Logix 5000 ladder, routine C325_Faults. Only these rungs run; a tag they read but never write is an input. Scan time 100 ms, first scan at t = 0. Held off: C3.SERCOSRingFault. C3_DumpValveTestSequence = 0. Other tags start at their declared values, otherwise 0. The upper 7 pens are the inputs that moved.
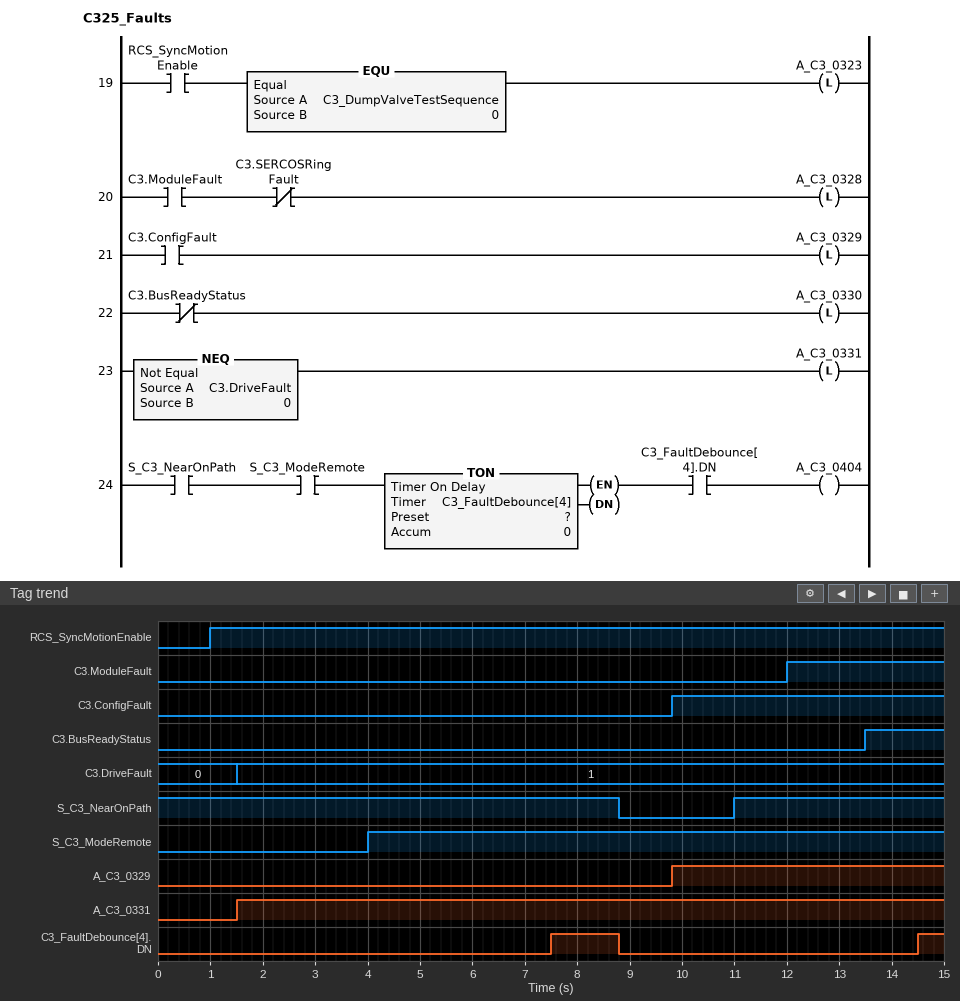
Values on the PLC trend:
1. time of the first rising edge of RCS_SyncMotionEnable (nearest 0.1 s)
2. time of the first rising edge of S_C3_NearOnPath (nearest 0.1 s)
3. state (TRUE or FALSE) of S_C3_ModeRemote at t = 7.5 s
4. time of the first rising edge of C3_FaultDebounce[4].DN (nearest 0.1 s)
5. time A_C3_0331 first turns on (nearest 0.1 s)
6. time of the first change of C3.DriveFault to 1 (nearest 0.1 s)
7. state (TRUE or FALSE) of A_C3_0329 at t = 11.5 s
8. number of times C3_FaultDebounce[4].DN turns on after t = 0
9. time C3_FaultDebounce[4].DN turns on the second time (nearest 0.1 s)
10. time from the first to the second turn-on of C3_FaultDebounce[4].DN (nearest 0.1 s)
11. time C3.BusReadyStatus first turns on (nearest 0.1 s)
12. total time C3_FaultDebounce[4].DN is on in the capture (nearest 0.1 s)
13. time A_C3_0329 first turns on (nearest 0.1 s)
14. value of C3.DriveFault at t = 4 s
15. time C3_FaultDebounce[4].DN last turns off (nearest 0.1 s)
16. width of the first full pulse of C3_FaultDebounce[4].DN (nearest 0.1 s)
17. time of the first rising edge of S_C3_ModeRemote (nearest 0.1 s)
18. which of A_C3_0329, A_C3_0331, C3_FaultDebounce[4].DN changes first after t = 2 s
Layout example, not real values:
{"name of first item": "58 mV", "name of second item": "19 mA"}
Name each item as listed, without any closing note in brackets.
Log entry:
{"time of the first rising edge of RCS_SyncMotionEnable": "1.0 s", "time of the first rising edge of S_C3_NearOnPath": "11.0 s", "state (TRUE or FALSE) of S_C3_ModeRemote at t = 7.5 s": "TRUE", "time of the first rising edge of C3_FaultDebounce[4].DN": "7.5 s", "time A_C3_0331 first turns on": "1.5 s", "time of the first change of C3.DriveFault to 1": "1.5 s", "state (TRUE or FALSE) of A_C3_0329 at t = 11.5 s": "TRUE", "number of times C3_FaultDebounce[4].DN turns on after t = 0": "2", "time C3_FaultDebounce[4].DN turns on the second time": "14.5 s", "time from the first to the second turn-on of C3_FaultDebounce[4].DN": "7.0 s", "time C3.BusReadyStatus first turns on": "13.5 s", "total time C3_FaultDebounce[4].DN is on in the capture": "1.8 s", "time A_C3_0329 first turns on": "9.8 s", "value of C3.DriveFault at t = 4 s": "1", "time C3_FaultDebounce[4].DN last turns off": "8.8 s", "width of the first full pulse of C3_FaultDebounce[4].DN": "1.3 s", "time of the first rising edge of S_C3_ModeRemote": "4.0 s", "which of A_C3_0329, A_C3_0331, C3_FaultDebounce[4].DN changes first after t = 2 s": "C3_FaultDebounce[4].DN"}
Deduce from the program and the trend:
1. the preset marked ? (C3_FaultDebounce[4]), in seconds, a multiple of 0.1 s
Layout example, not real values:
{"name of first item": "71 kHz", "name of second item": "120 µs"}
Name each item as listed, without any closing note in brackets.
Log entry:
{"the preset marked ? (C3_FaultDebounce[4]), in seconds, a multiple of 0.1 s": "3.5 s"}
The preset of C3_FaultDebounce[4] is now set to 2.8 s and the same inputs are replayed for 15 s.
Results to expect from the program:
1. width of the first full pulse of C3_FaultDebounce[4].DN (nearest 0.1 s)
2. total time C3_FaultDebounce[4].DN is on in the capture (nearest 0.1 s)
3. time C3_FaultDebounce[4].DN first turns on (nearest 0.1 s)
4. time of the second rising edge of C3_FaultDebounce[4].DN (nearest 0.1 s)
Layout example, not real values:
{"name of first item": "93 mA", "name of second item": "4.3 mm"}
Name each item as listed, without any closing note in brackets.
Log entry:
{"width of the first full pulse of C3_FaultDebounce[4].DN": "2.0 s", "total time C3_FaultDebounce[4].DN is on in the capture": "3.2 s", "time C3_FaultDebounce[4].DN first turns on": "6.8 s", "time of the second rising edge of C3_FaultDebounce[4].DN": "13.8 s"}
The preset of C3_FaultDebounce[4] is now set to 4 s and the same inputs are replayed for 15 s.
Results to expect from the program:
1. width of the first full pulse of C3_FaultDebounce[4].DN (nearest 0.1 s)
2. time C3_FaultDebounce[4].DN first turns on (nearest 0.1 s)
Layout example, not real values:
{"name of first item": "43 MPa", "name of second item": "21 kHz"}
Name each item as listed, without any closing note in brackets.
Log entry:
{"width of the first full pulse of C3_FaultDebounce[4].DN": "0.8 s", "time C3_FaultDebounce[4].DN first turns on": "8.0 s"}
